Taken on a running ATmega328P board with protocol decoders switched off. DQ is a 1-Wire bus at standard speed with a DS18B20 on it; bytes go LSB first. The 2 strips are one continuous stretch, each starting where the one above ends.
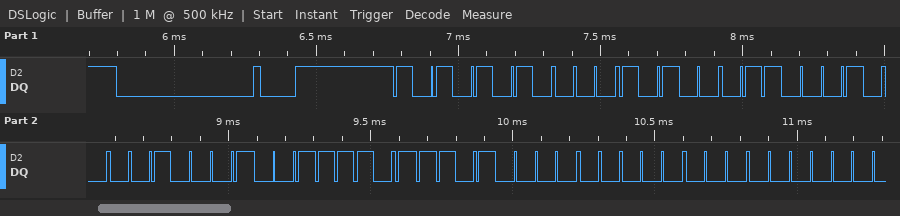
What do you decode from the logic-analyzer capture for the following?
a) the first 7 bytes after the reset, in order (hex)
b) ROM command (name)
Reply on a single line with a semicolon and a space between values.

55 28 46 88 BC 0B 00; Match ROM
